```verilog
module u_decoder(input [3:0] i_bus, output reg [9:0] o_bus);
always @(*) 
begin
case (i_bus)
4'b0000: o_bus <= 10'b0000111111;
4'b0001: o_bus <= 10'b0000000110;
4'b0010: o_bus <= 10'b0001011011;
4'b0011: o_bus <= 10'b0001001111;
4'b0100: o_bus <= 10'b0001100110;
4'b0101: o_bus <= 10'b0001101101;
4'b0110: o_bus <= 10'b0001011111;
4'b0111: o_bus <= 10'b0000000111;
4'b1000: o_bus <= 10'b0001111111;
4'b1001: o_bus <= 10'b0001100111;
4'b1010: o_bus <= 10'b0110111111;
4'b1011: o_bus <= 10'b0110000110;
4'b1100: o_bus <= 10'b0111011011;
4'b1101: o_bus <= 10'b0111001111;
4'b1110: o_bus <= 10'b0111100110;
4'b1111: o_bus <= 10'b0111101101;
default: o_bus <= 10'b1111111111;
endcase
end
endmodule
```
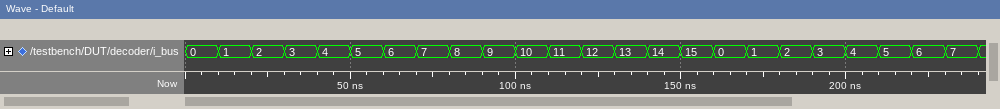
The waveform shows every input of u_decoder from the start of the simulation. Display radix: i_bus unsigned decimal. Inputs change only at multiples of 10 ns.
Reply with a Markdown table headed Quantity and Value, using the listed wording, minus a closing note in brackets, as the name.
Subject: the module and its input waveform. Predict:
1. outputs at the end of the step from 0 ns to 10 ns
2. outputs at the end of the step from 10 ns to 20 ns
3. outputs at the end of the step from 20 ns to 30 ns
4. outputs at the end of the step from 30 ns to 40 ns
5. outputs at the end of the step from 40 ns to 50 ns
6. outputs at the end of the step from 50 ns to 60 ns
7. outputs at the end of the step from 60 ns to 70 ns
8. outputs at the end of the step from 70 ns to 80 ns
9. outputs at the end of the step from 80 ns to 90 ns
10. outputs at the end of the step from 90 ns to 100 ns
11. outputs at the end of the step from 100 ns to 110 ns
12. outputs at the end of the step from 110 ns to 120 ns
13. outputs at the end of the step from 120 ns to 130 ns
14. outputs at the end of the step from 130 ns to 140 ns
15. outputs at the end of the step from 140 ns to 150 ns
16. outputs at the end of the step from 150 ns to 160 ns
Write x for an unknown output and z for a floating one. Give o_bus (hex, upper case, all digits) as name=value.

| Quantity | Value |
|---|---|
| outputs at the end of the step from 0 ns to 10 ns | o_bus=03F |
| outputs at the end of the step from 10 ns to 20 ns | o_bus=006 |
| outputs at the end of the step from 20 ns to 30 ns | o_bus=05B |
| outputs at the end of the step from 30 ns to 40 ns | o_bus=04F |
| outputs at the end of the step from 40 ns to 50 ns | o_bus=066 |
| outputs at the end of the step from 50 ns to 60 ns | o_bus=06D |
| outputs at the end of the step from 60 ns to 70 ns | o_bus=05F |
| outputs at the end of the step from 70 ns to 80 ns | o_bus=007 |
| outputs at the end of the step from 80 ns to 90 ns | o_bus=07F |
| outputs at the end of the step from 90 ns to 100 ns | o_bus=067 |
| outputs at the end of the step from 100 ns to 110 ns | o_bus=1BF |
| outputs at the end of the step from 110 ns to 120 ns | o_bus=186 |
| outputs at the end of the step from 120 ns to 130 ns | o_bus=1DB |
| outputs at the end of the step from 130 ns to 140 ns | o_bus=1CF |
| outputs at the end of the step from 140 ns to 150 ns | o_bus=1E6 |
| outputs at the end of the step from 150 ns to 160 ns | o_bus=1ED |
